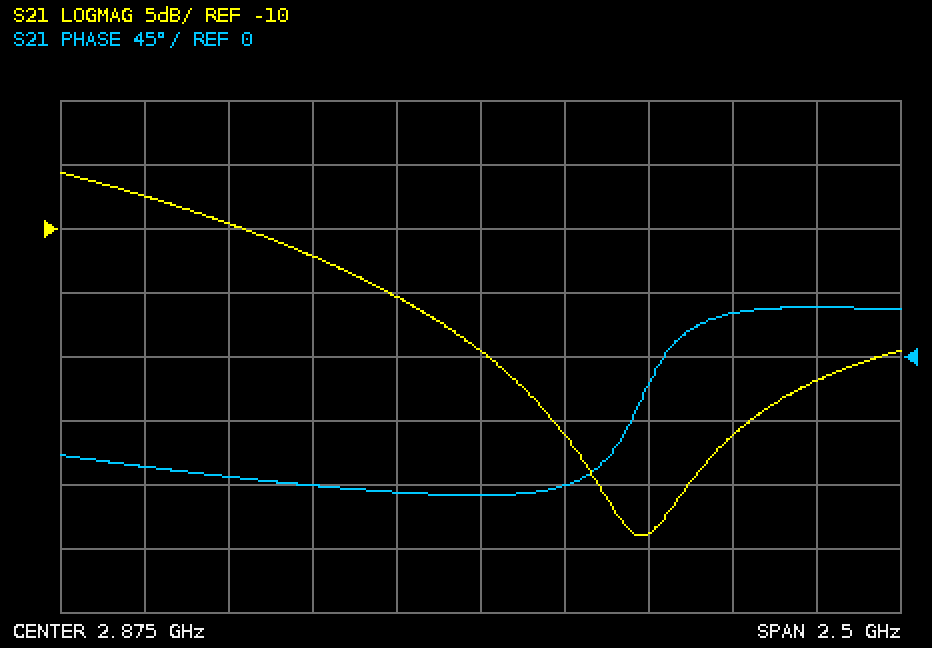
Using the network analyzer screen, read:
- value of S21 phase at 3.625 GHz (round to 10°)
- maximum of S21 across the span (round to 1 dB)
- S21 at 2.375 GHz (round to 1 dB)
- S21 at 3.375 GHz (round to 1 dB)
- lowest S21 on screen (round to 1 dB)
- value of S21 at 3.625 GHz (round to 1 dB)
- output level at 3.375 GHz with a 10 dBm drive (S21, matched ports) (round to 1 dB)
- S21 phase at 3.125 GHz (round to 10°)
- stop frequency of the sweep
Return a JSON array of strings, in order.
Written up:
["30°", "-6 dB", "-12 dB", "-34 dB", "-34 dB", "-26 dB", "-24 dBm", "-90°", "4.125 GHz"]
